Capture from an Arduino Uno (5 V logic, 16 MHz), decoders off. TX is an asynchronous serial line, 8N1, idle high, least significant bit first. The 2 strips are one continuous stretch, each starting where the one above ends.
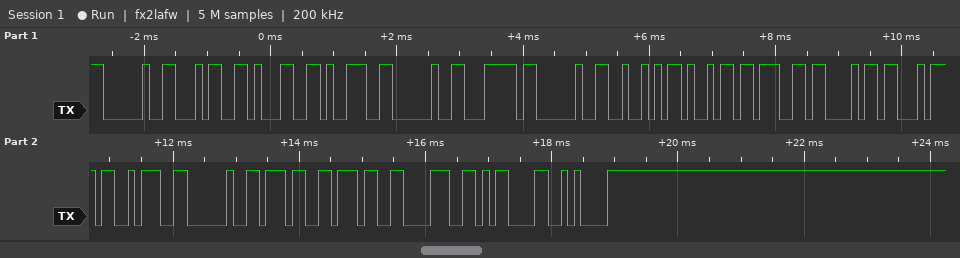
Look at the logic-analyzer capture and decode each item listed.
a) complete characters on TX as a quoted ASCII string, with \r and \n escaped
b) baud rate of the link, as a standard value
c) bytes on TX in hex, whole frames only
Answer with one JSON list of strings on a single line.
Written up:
["\" 419 | Right: 778\\r\\n\"", "9600 baud", "20 34 31 39 20 7C 20 52 69 67 68 74 3A 20 37 37 38 0D 0A"]
